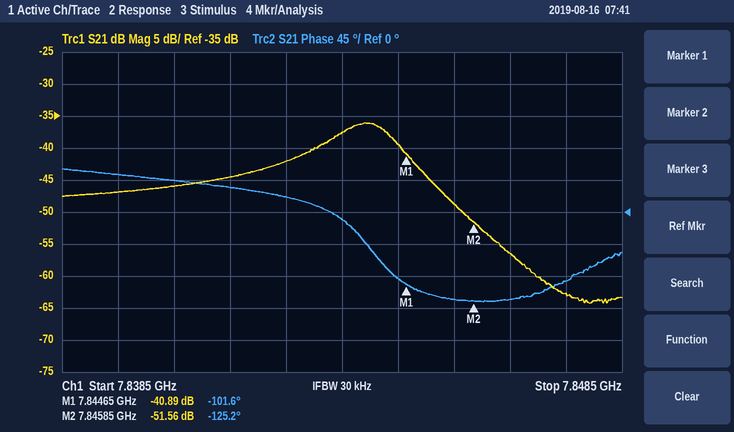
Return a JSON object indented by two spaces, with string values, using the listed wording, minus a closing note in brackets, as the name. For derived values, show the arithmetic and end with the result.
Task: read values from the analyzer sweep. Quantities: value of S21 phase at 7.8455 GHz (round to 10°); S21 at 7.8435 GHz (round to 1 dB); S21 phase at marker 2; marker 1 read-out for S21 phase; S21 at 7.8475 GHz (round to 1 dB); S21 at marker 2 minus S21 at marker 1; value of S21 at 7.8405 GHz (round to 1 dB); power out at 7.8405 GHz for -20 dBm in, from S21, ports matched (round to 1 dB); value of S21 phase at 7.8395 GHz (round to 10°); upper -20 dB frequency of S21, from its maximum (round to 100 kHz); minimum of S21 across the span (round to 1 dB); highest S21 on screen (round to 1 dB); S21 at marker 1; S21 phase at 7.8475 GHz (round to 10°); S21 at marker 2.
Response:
{
  "value of S21 phase at 7.8455 GHz": "-120°",
  "S21 at 7.8435 GHz": "-38 dB",
  "S21 phase at marker 2": "-125.2°",
  "marker 1 read-out for S21 phase": "-101.6°",
  "S21 at 7.8475 GHz": "-63 dB",
  "S21 at marker 2 minus S21 at marker 1": "-51.56 − (-40.89) = -10.67 dB",
  "value of S21 at 7.8405 GHz": "-46 dB",
  "power out at 7.8405 GHz for -20 dBm in, from S21, ports matched": "-20 dBm + (-46 dB) = -66 dBm",
  "value of S21 phase at 7.8395 GHz": "50°",
  "upper -20 dB frequency of S21, from its maximum": "7.8464 GHz",
  "minimum of S21 across the span": "-64 dB",
  "highest S21 on screen": "-36 dB",
  "S21 at marker 1": "-40.89 dB",
  "S21 phase at 7.8475 GHz": "-100°",
  "S21 at marker 2": "-51.56 dB"
}
